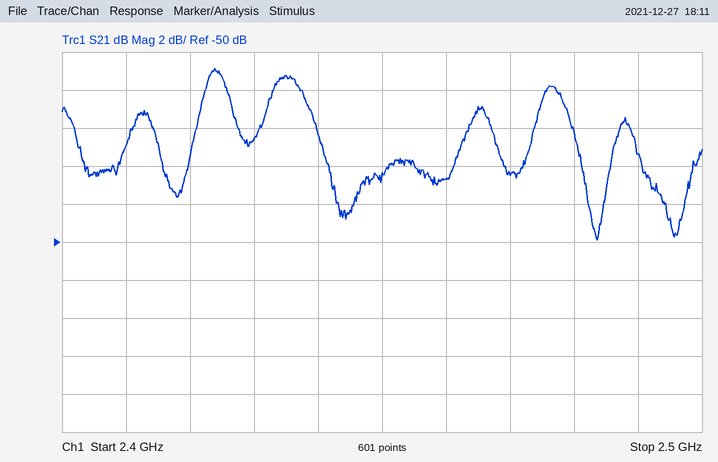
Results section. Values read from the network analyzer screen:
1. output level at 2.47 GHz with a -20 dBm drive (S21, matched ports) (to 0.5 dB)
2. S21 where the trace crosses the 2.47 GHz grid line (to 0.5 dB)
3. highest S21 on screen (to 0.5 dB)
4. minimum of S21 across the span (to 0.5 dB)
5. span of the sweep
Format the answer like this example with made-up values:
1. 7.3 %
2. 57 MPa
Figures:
1. -66.5 dBm
2. -46.5 dB
3. -41.0 dB
4. -50.0 dB
5. 100 MHz
